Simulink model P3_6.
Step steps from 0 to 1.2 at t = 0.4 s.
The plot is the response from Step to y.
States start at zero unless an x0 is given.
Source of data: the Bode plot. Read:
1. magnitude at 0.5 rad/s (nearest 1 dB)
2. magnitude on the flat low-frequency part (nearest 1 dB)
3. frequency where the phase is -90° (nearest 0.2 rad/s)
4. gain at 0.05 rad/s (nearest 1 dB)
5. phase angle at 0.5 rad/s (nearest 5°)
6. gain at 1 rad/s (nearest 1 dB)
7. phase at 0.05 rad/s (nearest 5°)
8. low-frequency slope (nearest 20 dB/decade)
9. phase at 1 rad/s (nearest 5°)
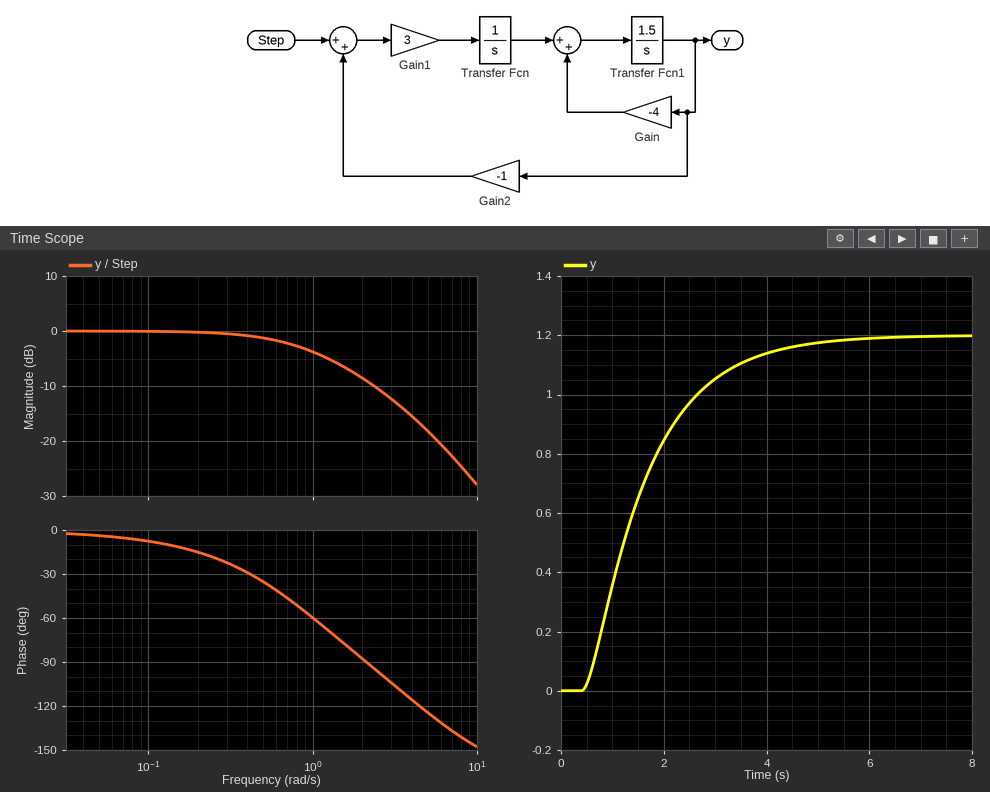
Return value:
-1 dB
0 dB
2.2 rad/s
0 dB
-35°
-4 dB
-5°
0 dB/decade
-60°
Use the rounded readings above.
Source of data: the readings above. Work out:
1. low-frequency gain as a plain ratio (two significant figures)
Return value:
1.0
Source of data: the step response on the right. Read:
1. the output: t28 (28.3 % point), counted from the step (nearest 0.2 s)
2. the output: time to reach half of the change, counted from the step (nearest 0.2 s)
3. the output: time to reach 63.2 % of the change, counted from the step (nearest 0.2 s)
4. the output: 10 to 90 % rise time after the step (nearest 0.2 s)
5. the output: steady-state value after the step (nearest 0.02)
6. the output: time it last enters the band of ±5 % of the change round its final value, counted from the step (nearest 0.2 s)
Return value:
0.6 s
1.0 s
1.4 s
2.6 s
1.20
3.6 s
